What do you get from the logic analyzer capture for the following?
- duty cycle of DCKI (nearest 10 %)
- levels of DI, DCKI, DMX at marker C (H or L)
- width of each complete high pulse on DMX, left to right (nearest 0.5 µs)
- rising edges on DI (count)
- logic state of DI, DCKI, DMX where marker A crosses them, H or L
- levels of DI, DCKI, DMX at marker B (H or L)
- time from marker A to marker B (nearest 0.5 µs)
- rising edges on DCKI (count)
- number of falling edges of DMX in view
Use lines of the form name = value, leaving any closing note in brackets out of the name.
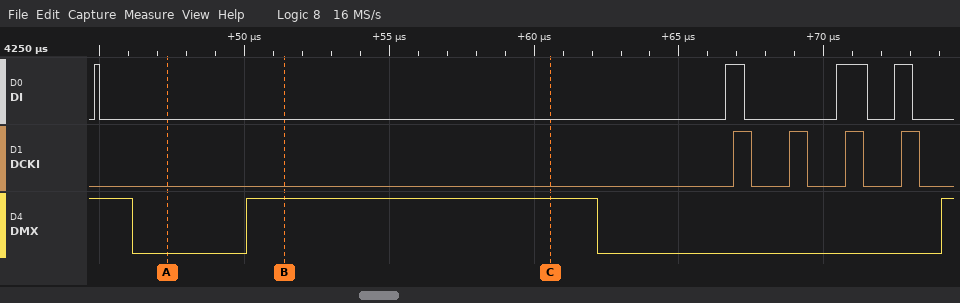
duty cycle of DCKI = 30 %
levels of DI, DCKI, DMX at marker C = DI=L, DCKI=L, DMX=H
width of each complete high pulse on DMX, left to right = 12 µs
rising edges on DI = 4
logic state of DI, DCKI, DMX where marker A crosses them, H or L = DI=L, DCKI=L, DMX=L
levels of DI, DCKI, DMX at marker B = DI=L, DCKI=L, DMX=H
time from marker A to marker B = 4 µs
rising edges on DCKI = 4
number of falling edges of DMX in view = 2
